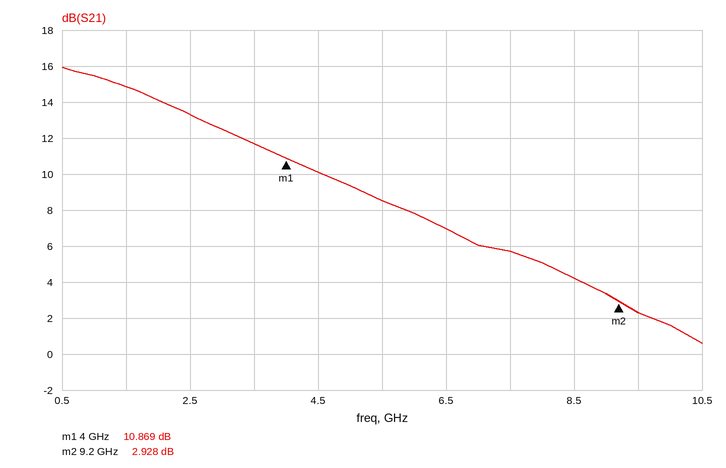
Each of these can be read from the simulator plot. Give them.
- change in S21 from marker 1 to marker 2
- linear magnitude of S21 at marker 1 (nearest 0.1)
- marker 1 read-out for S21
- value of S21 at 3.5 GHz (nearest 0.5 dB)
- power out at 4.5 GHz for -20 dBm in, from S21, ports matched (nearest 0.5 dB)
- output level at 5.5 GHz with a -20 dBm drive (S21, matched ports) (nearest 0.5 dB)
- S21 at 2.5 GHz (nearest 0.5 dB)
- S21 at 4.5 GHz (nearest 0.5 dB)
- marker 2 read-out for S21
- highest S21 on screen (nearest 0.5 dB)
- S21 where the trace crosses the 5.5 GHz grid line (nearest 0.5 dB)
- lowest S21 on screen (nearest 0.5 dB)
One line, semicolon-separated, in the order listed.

-7.941 dB; 3.5; 10.869 dB; 11.5 dB; -10.0 dBm; -11.5 dBm; 13.5 dB; 10.0 dB; 2.928 dB; 16.0 dB; 8.5 dB; 0.5 dB
